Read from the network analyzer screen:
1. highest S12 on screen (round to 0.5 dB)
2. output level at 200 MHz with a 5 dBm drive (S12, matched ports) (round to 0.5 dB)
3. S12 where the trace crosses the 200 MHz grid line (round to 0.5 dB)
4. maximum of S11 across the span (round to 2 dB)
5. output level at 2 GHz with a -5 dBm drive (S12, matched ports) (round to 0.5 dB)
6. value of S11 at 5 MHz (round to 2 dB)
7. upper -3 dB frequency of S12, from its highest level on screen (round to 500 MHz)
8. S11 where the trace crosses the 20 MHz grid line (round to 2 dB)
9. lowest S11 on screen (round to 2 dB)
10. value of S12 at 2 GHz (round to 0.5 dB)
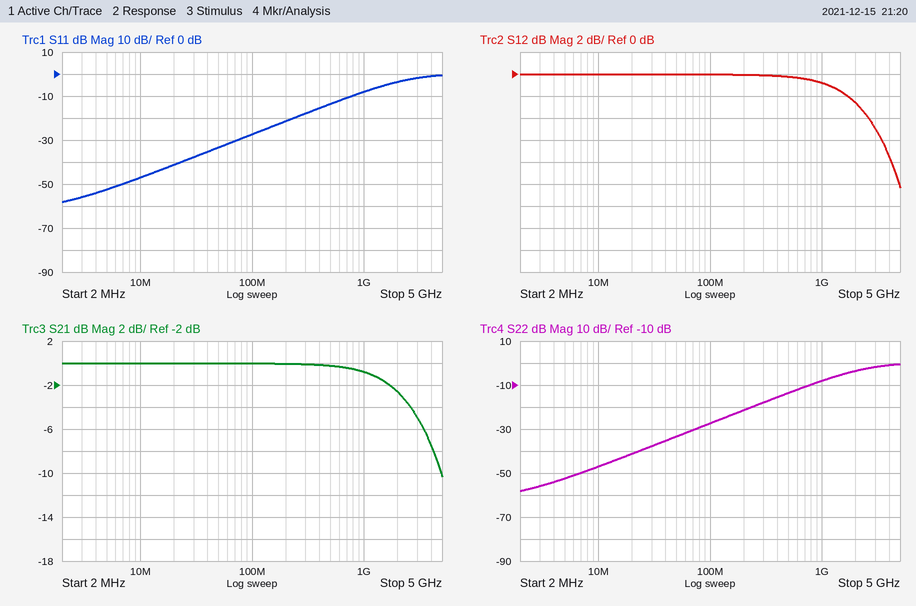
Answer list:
0.0 dB
5.0 dBm
0.0 dB
0 dB
-7.5 dBm
-52 dB
2.0 GHz
-42 dB
-58 dB
-2.5 dB
